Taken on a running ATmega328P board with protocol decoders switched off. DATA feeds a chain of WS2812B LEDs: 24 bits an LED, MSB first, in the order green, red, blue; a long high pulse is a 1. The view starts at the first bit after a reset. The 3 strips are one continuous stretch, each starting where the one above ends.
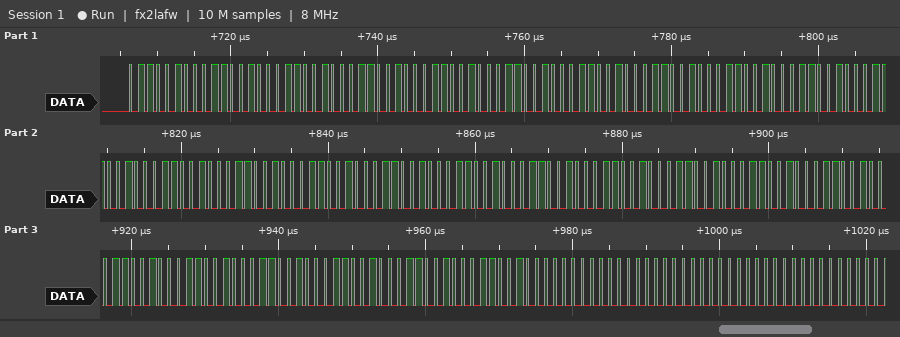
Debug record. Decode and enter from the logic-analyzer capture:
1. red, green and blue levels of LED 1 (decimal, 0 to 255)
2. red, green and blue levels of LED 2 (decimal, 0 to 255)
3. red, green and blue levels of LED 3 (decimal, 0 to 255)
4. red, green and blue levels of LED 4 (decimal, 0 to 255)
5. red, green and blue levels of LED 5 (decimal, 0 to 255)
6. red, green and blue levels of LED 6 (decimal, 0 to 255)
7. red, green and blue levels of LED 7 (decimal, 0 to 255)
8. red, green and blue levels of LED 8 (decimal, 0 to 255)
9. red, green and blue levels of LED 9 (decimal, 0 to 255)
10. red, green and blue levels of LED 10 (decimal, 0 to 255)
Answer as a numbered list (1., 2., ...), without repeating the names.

1. 100, 100, 100
2. 100, 100, 100
3. 100, 100, 100
4. 100, 100, 100
5. 100, 100, 100
6. 100, 100, 100
7. 100, 100, 100
8. 100, 100, 100
9. 100, 100, 100
10. 0, 0, 0
